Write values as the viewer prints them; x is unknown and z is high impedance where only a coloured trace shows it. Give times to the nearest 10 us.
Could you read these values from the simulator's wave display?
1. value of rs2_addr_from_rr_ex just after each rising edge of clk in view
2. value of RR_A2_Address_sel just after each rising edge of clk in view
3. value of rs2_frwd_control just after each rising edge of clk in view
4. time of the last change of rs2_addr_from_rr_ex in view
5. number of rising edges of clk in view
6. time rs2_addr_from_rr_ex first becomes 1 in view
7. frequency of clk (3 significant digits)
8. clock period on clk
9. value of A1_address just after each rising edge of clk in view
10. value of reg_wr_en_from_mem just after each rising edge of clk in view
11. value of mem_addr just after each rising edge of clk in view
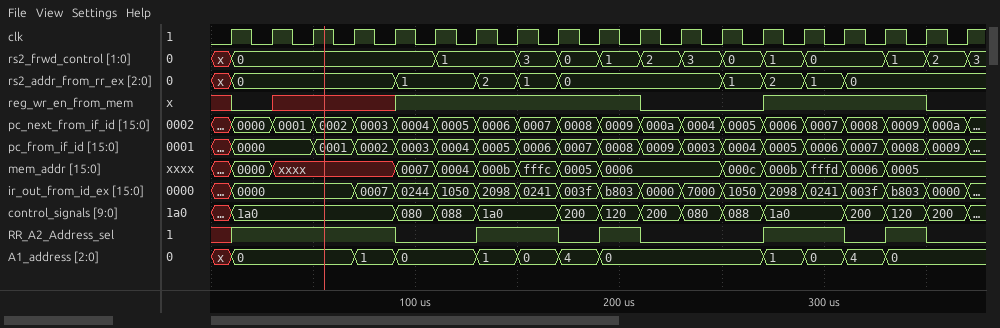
0, 0, 0, 0, 1, 1, 2, 1, 0, 0, 0, 0, 1, 2, 1, 0, 0, 0, 0
1 1 1 1 0 0 1 1 0 1 0 0 0 1 1 0 1 0 0
0, 0, 0, 0, 0, 1, 1, 3, 0, 1, 2, 3, 0, 1, 0, 0, 1, 2, 3
310 us
19
90 us
50.0 kHz
20 us
0, 0, 0, 1, 0, 0, 1, 0, 4, 0, 0, 0, 0, 1, 0, 4, 0, 0, 0
0 x x x 1 1 1 1 1 1 0 0 0 1 1 1 1 0 0
0000, xxxx, xxxx, xxxx, 0007, 0004, 000b, fffc, 0005, 0006, 0006, 0006, 000c, 000b, fffd, 0006, 0005, 0005, 0005
